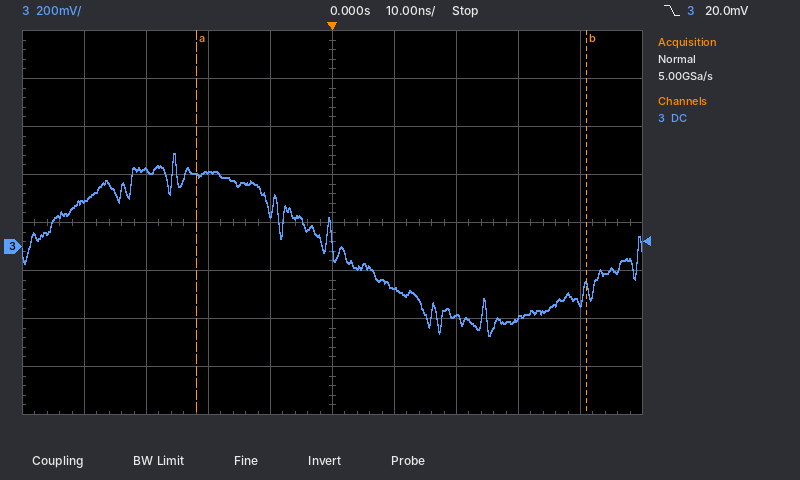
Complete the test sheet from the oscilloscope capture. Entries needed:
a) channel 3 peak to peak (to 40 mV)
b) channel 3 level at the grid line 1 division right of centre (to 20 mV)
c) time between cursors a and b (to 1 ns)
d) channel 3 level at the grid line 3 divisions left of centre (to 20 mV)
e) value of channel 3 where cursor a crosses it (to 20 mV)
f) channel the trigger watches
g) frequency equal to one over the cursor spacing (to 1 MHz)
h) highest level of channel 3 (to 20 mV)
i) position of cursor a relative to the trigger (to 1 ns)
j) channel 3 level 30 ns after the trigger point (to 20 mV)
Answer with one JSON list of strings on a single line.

["760 mV", "-180 mV", "63 ns", "320 mV", "300 mV", "channel 3", "16 MHz", "380 mV", "-22 ns", "-300 mV"]
